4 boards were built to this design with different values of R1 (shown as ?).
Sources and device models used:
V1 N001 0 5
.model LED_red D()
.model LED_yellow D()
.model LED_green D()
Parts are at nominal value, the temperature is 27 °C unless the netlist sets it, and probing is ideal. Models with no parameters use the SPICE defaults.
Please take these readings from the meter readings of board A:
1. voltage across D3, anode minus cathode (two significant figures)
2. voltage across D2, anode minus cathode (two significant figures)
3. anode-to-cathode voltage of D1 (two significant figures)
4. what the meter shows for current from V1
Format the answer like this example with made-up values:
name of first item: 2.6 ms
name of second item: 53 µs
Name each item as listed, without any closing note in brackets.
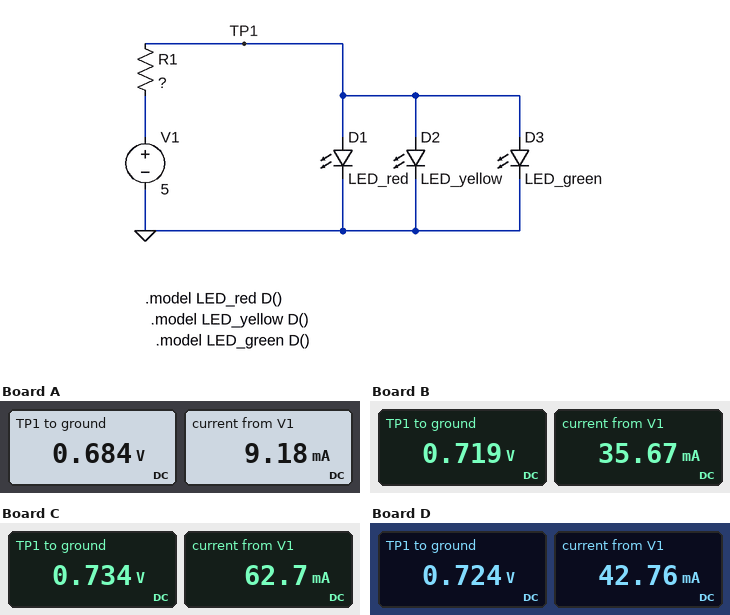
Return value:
voltage across D3, anode minus cathode: 680 mV
voltage across D2, anode minus cathode: 680 mV
anode-to-cathode voltage of D1: 680 mV
what the meter shows for current from V1: 9.18 mA
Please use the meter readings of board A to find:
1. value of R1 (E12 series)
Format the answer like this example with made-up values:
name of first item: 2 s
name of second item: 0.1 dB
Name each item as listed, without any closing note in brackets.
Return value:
value of R1: 470 Ω
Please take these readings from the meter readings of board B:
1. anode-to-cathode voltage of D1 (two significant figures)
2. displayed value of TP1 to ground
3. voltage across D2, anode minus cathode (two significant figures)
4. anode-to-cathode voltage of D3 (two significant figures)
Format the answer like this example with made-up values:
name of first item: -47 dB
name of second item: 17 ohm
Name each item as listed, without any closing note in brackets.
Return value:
anode-to-cathode voltage of D1: 720 mV
displayed value of TP1 to ground: 0.719 V
voltage across D2, anode minus cathode: 720 mV
anode-to-cathode voltage of D3: 720 mV
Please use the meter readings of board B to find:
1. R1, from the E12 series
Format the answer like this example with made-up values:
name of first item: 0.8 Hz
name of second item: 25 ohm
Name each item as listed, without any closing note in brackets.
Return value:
R1, from the E12 series: 120 Ω
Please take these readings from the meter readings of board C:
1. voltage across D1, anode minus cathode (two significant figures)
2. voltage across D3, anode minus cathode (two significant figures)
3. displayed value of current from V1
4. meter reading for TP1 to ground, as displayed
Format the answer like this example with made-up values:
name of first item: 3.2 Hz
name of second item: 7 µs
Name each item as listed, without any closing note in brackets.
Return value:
voltage across D1, anode minus cathode: 730 mV
voltage across D3, anode minus cathode: 730 mV
displayed value of current from V1: 62.7 mA
meter reading for TP1 to ground, as displayed: 0.734 V
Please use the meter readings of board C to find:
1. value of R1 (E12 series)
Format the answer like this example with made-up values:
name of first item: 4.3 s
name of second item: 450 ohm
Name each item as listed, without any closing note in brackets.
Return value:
value of R1: 68 Ω
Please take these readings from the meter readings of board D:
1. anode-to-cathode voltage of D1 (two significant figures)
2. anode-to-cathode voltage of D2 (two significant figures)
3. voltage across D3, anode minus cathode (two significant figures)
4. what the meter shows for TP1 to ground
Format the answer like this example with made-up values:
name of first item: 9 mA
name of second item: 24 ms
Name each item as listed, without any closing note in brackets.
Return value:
anode-to-cathode voltage of D1: 720 mV
anode-to-cathode voltage of D2: 720 mV
voltage across D3, anode minus cathode: 720 mV
what the meter shows for TP1 to ground: 0.724 V
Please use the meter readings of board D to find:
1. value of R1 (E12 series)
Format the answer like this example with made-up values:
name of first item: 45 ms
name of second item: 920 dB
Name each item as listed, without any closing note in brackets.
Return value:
value of R1: 100 Ω
